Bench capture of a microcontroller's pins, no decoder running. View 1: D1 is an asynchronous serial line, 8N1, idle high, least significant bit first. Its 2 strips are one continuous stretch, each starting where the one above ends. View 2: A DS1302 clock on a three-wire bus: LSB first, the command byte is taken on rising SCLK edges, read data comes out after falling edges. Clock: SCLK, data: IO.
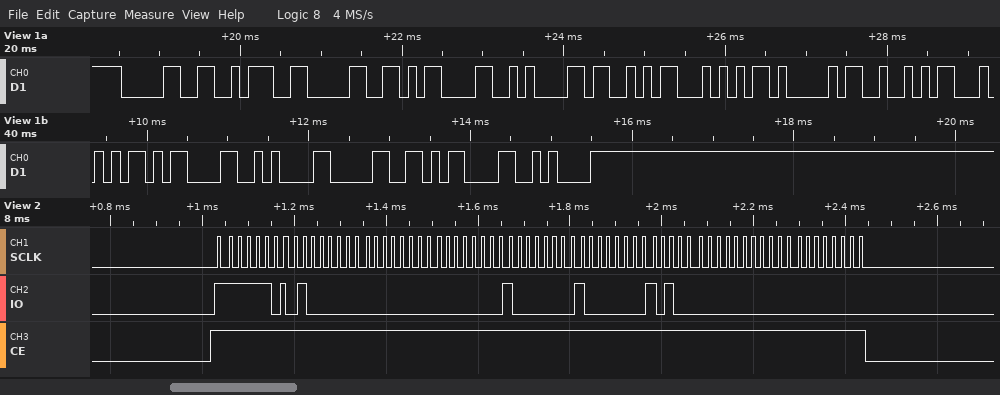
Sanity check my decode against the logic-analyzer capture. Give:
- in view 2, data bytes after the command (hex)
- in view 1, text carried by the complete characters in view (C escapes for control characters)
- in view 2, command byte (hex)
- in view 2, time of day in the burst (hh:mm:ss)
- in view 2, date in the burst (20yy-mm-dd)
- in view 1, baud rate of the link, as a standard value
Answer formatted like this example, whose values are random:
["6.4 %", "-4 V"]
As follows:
["02 00 00 01 01 05 00 00", "\"0:0\\r\\nSTART\\r\\n0\\r\\n\"", "0xBF", "00:00:02", "2000-01-01", "9600 baud"]
